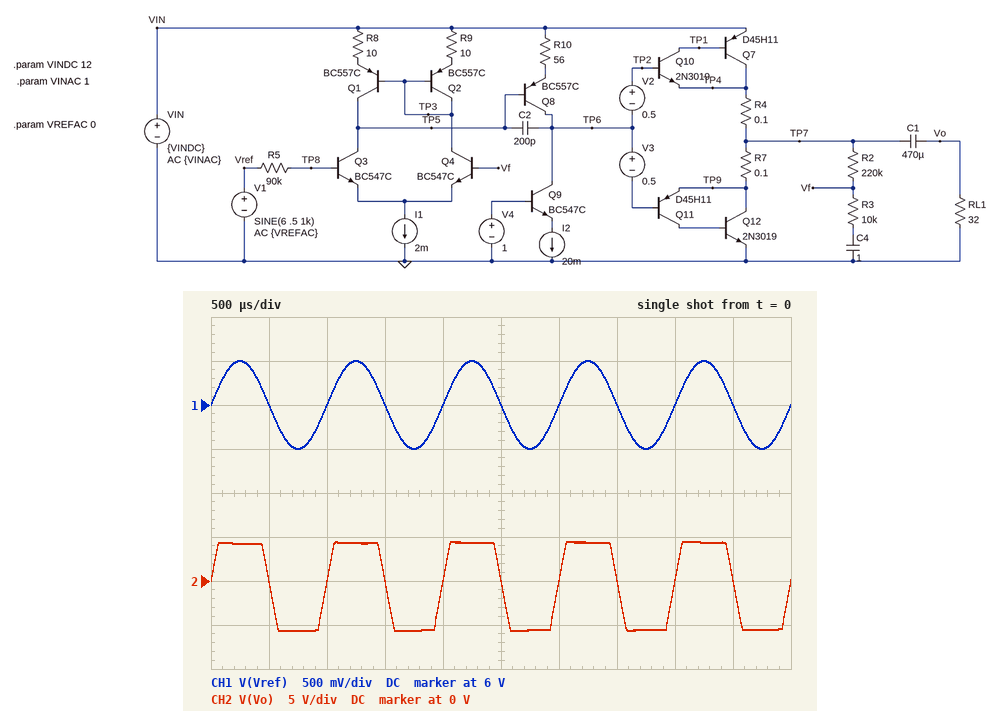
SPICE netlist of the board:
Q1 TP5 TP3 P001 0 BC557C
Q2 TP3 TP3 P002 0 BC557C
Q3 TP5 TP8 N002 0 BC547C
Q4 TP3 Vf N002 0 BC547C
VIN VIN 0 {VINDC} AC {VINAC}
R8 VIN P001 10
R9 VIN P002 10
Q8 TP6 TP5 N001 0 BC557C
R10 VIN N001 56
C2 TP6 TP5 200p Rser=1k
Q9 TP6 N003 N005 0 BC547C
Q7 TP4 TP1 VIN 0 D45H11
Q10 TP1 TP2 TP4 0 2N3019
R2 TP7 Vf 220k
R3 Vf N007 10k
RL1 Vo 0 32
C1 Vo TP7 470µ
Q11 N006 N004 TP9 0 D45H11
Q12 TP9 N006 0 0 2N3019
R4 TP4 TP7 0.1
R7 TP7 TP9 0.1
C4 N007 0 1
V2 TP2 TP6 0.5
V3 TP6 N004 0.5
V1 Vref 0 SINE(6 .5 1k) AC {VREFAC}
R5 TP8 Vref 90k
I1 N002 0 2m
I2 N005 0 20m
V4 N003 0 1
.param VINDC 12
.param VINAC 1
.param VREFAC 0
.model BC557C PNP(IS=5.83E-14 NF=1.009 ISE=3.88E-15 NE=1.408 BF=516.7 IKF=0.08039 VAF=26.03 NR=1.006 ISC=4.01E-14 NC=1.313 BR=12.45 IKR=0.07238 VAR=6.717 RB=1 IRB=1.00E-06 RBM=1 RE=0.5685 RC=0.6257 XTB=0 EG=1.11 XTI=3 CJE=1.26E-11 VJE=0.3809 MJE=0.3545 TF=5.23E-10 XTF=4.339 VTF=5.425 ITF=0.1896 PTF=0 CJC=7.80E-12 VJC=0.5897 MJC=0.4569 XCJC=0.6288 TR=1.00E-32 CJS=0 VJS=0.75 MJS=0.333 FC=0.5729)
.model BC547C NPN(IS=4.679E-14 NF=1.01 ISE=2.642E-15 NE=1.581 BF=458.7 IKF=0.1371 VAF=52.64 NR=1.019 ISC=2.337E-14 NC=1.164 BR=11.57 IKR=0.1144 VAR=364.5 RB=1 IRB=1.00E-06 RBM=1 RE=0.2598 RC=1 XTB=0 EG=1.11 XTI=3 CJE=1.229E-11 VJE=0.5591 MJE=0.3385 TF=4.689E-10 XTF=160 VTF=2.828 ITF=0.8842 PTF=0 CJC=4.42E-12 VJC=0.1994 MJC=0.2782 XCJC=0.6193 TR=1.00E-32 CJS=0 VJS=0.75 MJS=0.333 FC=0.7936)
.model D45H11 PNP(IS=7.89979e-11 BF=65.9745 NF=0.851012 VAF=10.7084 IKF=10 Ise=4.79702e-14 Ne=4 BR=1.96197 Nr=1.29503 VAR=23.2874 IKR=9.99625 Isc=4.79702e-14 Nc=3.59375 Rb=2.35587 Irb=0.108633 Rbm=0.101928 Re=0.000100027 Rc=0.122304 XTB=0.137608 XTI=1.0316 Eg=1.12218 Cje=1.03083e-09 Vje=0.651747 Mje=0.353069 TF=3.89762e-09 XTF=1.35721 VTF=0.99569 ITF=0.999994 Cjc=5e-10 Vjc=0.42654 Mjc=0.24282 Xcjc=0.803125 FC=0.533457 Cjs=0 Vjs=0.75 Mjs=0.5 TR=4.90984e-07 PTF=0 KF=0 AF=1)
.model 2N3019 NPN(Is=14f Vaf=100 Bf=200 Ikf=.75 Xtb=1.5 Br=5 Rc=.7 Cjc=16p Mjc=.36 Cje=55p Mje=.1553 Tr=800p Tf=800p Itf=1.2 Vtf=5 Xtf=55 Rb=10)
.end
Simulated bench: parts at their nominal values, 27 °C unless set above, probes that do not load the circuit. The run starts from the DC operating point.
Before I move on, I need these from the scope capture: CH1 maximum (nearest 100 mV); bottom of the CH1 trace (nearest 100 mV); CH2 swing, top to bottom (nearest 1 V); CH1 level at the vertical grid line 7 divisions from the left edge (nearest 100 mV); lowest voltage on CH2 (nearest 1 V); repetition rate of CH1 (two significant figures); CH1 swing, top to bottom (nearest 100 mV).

6.5 V
5.5 V
10 V
6.0 V
-6 V
1.0 kHz
1.0 V
